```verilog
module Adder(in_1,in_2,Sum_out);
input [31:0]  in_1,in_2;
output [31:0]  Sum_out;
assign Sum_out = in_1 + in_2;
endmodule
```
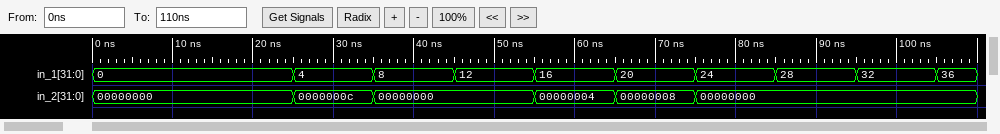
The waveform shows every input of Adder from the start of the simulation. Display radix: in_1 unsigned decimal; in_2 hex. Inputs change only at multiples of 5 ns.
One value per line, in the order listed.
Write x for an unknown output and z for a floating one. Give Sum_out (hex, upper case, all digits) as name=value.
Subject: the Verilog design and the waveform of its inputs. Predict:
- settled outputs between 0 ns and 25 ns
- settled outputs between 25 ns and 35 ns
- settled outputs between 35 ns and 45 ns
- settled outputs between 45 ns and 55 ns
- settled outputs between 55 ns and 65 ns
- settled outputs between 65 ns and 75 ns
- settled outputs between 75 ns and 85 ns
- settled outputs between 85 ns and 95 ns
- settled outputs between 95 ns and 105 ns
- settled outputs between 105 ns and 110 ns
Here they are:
Sum_out=00000000
Sum_out=00000010
Sum_out=00000008
Sum_out=0000000C
Sum_out=00000014
Sum_out=0000001C
Sum_out=00000018
Sum_out=0000001C
Sum_out=00000020
Sum_out=00000024
